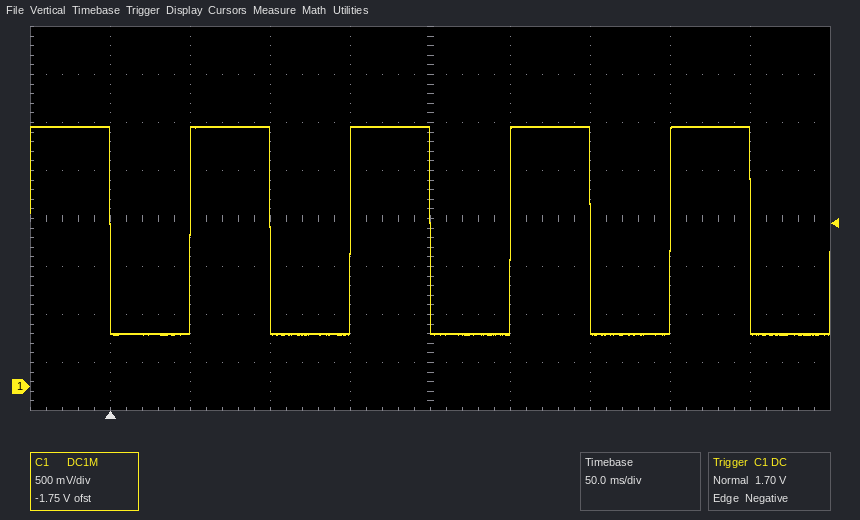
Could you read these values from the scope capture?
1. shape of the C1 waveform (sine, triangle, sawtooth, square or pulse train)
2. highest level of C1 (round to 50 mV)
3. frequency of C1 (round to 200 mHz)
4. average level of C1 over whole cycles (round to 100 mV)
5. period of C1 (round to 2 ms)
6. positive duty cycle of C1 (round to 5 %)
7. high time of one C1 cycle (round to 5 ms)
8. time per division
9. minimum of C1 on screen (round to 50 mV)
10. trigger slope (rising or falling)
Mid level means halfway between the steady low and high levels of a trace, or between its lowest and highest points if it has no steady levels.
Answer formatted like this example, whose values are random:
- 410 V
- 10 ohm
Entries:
- square
- 2.70 V
- 10.0 Hz
- 1.6 V
- 100 ms
- 50 %
- 50 ms
- 50 ms
- 550 mV
- falling
